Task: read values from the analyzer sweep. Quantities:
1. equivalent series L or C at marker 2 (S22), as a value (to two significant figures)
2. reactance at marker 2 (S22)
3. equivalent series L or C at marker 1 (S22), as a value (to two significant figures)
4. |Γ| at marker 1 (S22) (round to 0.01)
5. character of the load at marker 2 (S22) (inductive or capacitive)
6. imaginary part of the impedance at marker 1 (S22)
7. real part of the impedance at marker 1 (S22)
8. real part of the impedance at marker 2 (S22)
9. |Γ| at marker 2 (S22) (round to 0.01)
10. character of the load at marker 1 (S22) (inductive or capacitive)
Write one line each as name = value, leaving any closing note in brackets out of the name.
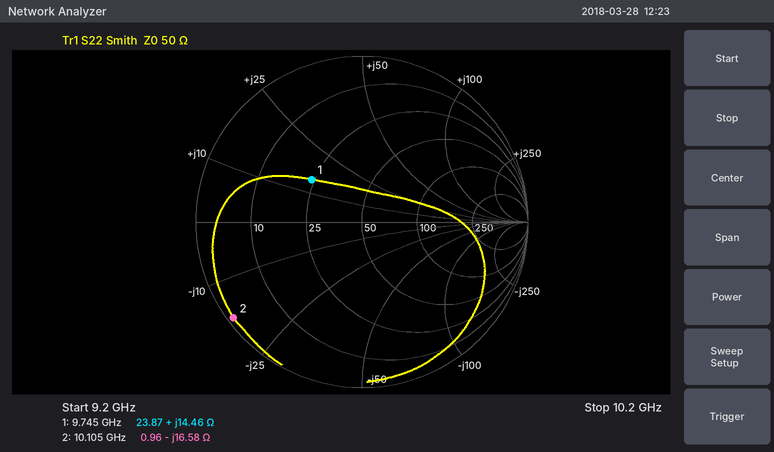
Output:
equivalent series L or C at marker 2 (S22), as a value = 950 fF
reactance at marker 2 = -16.58 Ω
equivalent series L or C at marker 1 (S22), as a value = 240 pH
|Γ| at marker 1 (S22) = 0.40
character of the load at marker 2 (S22) = capacitive
imaginary part of the impedance at marker 1 = +14.46 Ω
real part of the impedance at marker 1 = 23.87 Ω
real part of the impedance at marker 2 = 0.96 Ω
|Γ| at marker 2 (S22) = 0.97
character of the load at marker 1 (S22) = inductive
